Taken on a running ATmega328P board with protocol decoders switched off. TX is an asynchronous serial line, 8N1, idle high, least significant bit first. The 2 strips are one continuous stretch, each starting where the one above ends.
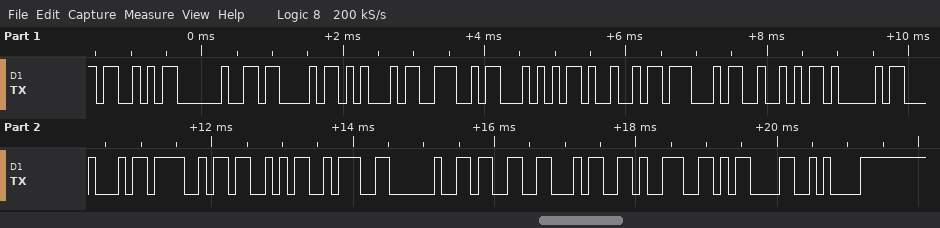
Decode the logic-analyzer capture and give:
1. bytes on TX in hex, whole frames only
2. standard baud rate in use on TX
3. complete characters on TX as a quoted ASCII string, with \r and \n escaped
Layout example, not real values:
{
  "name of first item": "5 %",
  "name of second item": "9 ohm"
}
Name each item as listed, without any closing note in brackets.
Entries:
{
  "bytes on TX in hex, whole frames only": "53 20 43 45 4E 54 49 47 52 41 44 4F 53 3A 20 33 34 39 0D 0A",
  "standard baud rate in use on TX": "9600 baud",
  "complete characters on TX as a quoted ASCII string, with \\r and \\n escaped": "\"S CENTIGRADOS: 349\\r\\n\""
}
